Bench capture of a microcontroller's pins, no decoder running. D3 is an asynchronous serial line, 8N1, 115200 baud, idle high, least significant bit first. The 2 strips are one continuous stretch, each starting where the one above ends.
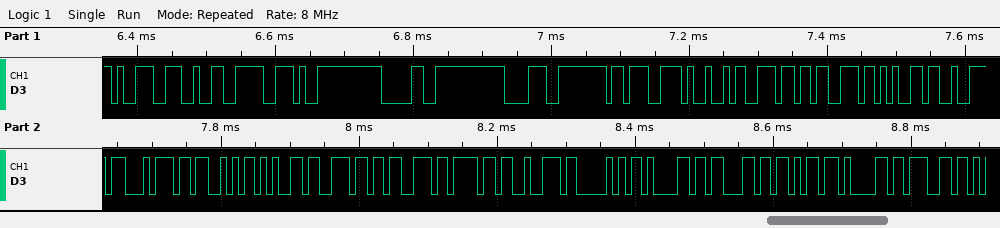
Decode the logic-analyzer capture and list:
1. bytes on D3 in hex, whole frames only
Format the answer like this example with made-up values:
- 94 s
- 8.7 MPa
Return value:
- 39 32 2E 30 38 3B 49 6E 73 65 72 74 53 65 6E 73 6F 72 50 61 63 6B 61 67
